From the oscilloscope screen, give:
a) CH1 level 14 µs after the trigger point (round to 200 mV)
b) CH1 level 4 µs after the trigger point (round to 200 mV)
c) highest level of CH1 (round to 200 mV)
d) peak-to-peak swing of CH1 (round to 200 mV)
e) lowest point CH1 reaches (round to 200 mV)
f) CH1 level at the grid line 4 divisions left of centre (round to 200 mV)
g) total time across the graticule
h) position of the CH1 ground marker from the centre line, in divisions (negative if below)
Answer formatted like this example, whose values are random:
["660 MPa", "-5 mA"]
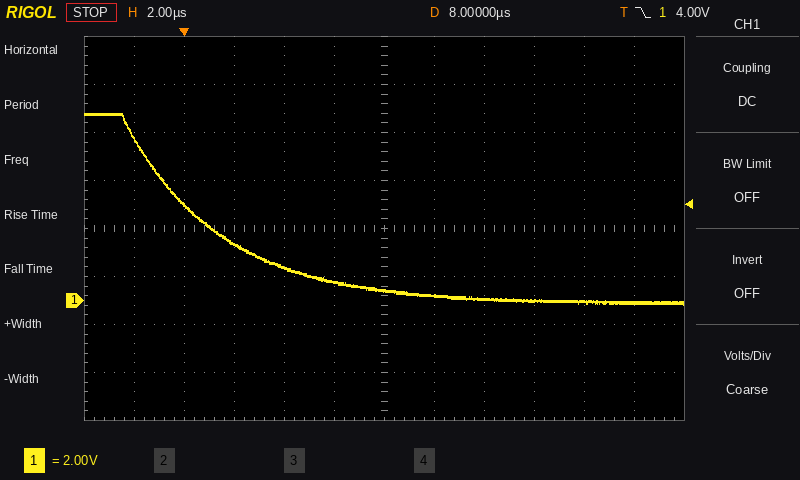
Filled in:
["0.0 V", "1.4 V", "7.8 V", "8.0 V", "-200 mV", "4.0 V", "24 µs", "-1.5 div"]
